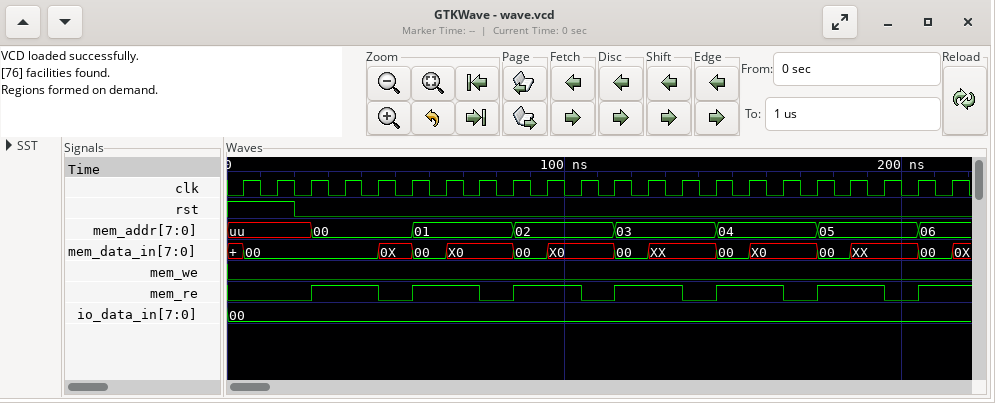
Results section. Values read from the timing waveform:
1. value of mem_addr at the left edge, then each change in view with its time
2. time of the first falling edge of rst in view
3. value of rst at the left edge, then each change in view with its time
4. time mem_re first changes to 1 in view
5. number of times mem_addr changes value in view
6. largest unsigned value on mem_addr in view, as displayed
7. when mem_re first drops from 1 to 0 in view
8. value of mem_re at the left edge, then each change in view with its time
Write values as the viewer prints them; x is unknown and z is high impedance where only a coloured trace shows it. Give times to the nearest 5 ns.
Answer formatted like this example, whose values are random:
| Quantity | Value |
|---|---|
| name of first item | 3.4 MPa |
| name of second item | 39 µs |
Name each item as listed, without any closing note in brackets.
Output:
| Quantity | Value |
|---|---|
| value of mem_addr at the left edge, then each change in view with its time | uu, 00 at 25 ns, 01 at 55 ns, 02 at 85 ns, 03 at 115 ns, 04 at 145 ns, 05 at 175 ns, 06 at 205 ns |
| time of the first falling edge of rst in view | 20 ns |
| value of rst at the left edge, then each change in view with its time | 1, 0 at 20 ns |
| time mem_re first changes to 1 in view | 25 ns |
| number of times mem_addr changes value in view | 7 |
| largest unsigned value on mem_addr in view, as displayed | 06 |
| when mem_re first drops from 1 to 0 in view | 45 ns |
| value of mem_re at the left edge, then each change in view with its time | 0, 1 at 25 ns, 0 at 45 ns, 1 at 55 ns, 0 at 75 ns, 1 at 85 ns, 0 at 105 ns, 1 at 115 ns, 0 at 135 ns, 1 at 145 ns, 0 at 165 ns, 1 at 175 ns, 0 at 195 ns, 1 at 205 ns |
